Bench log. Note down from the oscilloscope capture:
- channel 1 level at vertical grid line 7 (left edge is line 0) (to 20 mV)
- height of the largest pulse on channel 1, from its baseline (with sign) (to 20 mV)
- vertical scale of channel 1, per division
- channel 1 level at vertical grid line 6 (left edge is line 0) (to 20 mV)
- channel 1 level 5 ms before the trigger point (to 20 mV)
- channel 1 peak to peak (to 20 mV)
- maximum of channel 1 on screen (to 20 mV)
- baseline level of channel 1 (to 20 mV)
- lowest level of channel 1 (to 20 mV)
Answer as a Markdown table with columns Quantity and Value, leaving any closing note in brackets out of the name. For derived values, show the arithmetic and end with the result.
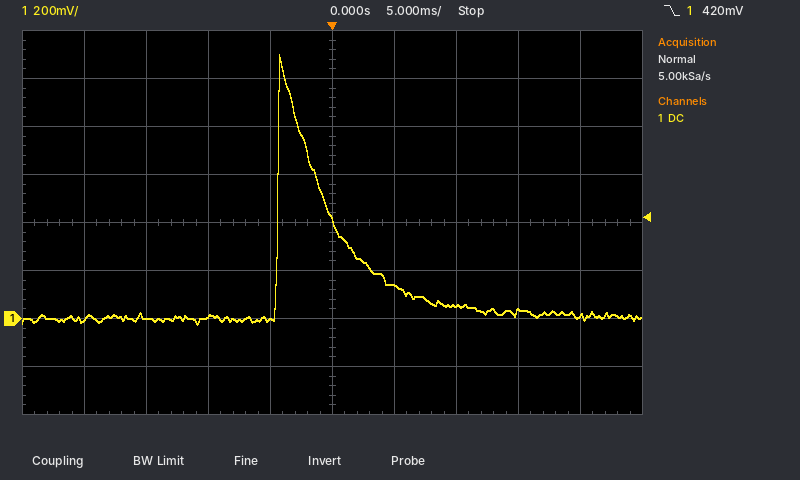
| Quantity | Value |
|---|---|
| channel 1 level at vertical grid line 7 (left edge is line 0) | 60 mV |
| height of the largest pulse on channel 1, from its baseline (with sign) | 1.10 V − (0 mV) = +1.10 V |
| vertical scale of channel 1, per division | 200 mV |
| channel 1 level at vertical grid line 6 (left edge is line 0) | 140 mV |
| channel 1 level 5 ms before the trigger point | 0 mV |
| channel 1 peak to peak | 1.10 V − (-20 mV) = 1.12 V |
| maximum of channel 1 on screen | 1.10 V |
| baseline level of channel 1 | 0 mV |
| lowest level of channel 1 | -20 mV |
